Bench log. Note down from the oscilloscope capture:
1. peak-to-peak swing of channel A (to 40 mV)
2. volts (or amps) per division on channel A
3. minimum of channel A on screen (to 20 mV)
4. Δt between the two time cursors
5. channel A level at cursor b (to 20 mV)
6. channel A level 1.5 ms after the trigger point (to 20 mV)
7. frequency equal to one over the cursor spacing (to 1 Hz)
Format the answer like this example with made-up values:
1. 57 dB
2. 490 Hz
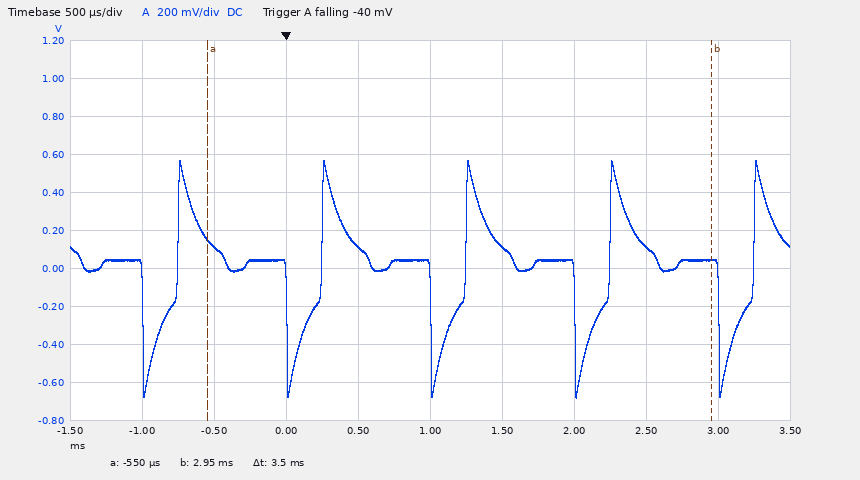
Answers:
1. 1.24 V
2. 200 mV
3. -680 mV
4. 3.5 ms
5. 40 mV
6. 120 mV
7. 286 Hz
